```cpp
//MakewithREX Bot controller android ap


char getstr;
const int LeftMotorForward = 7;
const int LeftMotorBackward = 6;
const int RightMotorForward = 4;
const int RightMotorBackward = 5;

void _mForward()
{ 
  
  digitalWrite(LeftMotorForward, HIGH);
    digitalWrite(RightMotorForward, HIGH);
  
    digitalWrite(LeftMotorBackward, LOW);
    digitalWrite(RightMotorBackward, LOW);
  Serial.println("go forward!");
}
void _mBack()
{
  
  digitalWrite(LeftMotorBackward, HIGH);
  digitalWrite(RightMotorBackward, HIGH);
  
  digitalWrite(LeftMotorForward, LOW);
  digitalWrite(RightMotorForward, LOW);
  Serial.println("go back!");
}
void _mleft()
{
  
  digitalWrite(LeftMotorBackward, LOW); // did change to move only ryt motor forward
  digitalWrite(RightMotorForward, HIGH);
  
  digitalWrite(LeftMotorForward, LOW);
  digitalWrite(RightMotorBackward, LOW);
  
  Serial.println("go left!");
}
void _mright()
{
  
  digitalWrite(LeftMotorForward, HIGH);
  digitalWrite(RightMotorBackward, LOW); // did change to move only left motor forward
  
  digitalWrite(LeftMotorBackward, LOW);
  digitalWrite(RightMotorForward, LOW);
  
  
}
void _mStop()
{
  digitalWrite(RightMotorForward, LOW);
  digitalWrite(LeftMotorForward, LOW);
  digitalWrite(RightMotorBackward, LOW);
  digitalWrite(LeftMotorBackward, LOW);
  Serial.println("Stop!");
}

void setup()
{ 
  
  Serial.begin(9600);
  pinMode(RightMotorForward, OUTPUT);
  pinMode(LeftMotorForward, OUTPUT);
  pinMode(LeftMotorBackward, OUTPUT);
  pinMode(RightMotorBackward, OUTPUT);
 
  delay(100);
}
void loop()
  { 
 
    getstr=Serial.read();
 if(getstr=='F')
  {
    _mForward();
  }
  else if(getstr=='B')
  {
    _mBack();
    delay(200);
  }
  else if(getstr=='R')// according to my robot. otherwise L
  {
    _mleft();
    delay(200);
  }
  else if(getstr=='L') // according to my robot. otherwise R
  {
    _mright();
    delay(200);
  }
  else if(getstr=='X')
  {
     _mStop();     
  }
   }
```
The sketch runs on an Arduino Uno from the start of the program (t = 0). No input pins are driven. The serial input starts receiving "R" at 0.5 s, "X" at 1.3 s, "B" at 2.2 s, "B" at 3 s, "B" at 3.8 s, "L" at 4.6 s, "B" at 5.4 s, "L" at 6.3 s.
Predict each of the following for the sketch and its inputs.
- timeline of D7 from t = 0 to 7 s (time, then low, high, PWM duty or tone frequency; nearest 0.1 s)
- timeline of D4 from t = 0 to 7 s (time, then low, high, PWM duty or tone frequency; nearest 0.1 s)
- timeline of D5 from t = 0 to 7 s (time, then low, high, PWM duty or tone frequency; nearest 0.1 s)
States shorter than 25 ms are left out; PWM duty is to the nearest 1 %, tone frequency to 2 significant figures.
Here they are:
0 s low; 4.6 s high; 5.4 s low; 6.3 s high
0 s low; 0.5 s high; 1.3 s low
0 s low; 2.2 s high; 4.6 s low; 5.4 s high; 6.3 s low
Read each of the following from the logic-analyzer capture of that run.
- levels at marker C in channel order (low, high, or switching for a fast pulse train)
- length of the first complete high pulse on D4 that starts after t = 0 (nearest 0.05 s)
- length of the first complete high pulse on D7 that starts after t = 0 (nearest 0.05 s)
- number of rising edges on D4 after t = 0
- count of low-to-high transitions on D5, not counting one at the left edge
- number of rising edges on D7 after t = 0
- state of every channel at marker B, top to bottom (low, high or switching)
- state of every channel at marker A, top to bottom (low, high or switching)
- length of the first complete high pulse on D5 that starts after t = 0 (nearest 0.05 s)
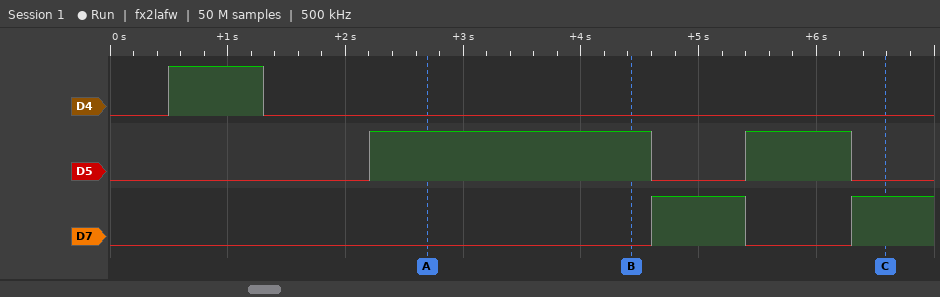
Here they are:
D4 low, D5 low, D7 high
0.80 s
0.80 s
1
2
2
D4 low, D5 high, D7 low
D4 low, D5 high, D7 low
2.40 s
